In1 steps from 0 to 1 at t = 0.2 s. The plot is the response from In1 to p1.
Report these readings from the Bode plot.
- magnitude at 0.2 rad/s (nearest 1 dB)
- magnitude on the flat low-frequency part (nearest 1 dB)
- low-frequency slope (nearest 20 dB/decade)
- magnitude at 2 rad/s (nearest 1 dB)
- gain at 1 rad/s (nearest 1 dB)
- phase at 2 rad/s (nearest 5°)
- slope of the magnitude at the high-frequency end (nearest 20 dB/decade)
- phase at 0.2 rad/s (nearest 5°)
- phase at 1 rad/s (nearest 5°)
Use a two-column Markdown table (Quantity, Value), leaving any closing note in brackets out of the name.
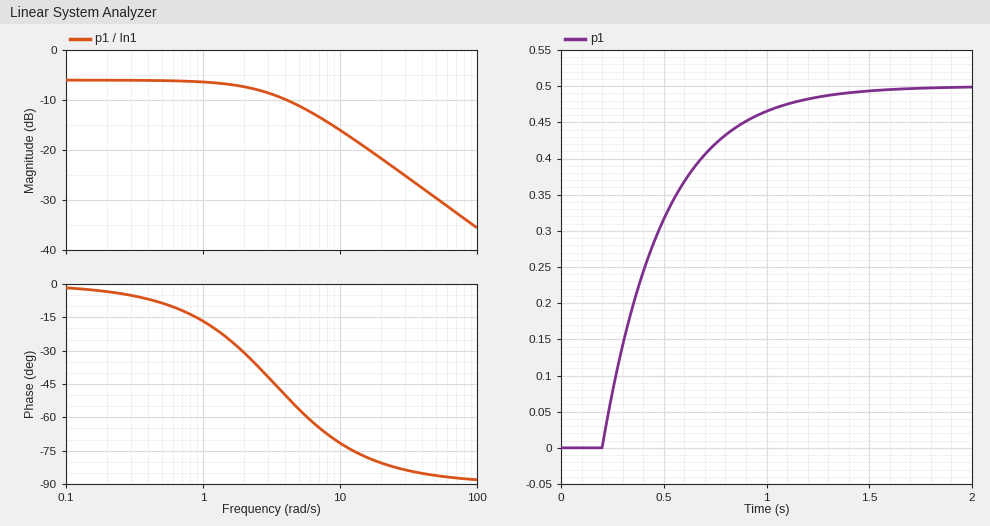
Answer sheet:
| Quantity | Value |
|---|---|
| magnitude at 0.2 rad/s | -6 dB |
| magnitude on the flat low-frequency part | -6 dB |
| low-frequency slope | 0 dB/decade |
| magnitude at 2 rad/s | -7 dB |
| gain at 1 rad/s | -6 dB |
| phase at 2 rad/s | -30° |
| slope of the magnitude at the high-frequency end | -20 dB/decade |
| phase at 0.2 rad/s | -5° |
| phase at 1 rad/s | -15° |
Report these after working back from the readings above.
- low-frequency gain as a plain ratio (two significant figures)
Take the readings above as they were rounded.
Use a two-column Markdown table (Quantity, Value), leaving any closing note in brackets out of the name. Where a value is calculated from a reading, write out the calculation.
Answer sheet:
| Quantity | Value |
|---|---|
| low-frequency gain as a plain ratio | 10^(-6 / 20) = 0.50 |
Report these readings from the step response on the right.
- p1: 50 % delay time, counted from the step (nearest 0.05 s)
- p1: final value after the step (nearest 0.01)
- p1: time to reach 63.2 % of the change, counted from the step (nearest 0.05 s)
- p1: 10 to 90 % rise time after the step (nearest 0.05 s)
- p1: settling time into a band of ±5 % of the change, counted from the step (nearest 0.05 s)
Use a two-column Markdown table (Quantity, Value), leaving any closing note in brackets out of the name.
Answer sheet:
| Quantity | Value |
|---|---|
| p1: 50 % delay time, counted from the step | 0.20 s |
| p1: final value after the step | 0.50 |
| p1: time to reach 63.2 % of the change, counted from the step | 0.30 s |
| p1: 10 to 90 % rise time after the step | 0.65 s |
| p1: settling time into a band of ±5 % of the change, counted from the step | 0.90 s |
